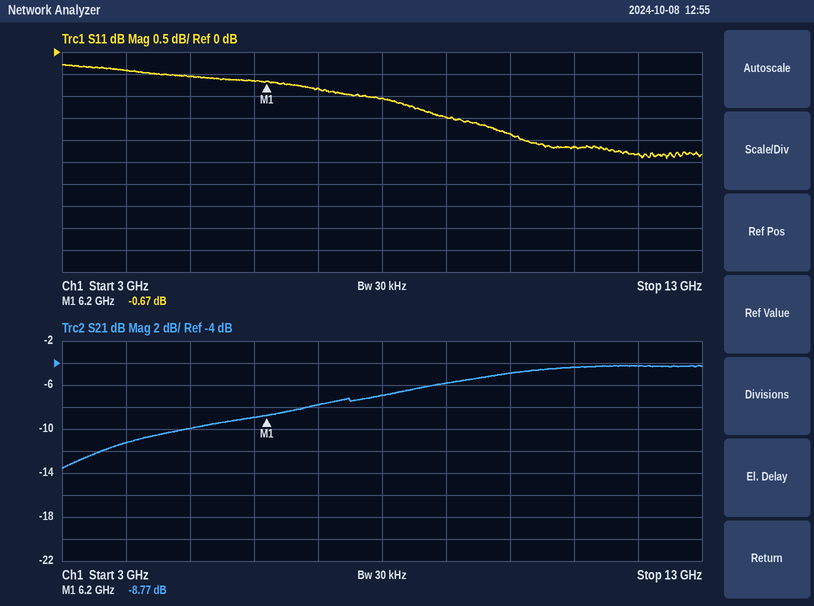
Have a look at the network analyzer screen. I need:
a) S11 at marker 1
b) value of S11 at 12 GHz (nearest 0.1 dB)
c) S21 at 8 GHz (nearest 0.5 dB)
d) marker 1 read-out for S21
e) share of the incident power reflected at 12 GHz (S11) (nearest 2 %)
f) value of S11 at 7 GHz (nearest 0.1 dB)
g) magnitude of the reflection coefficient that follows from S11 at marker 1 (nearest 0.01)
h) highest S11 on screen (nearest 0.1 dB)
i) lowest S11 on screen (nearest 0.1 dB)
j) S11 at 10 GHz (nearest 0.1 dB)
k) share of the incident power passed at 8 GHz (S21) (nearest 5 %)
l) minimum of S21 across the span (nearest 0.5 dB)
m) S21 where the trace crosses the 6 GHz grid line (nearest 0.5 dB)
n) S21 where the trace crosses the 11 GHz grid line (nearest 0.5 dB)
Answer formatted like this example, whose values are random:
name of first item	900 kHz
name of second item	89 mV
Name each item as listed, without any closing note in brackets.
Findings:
S11 at marker 1	-0.67 dB
value of S11 at 12 GHz	-2.3 dB
S21 at 8 GHz	-7.0 dB
marker 1 read-out for S21	-8.77 dB
share of the incident power reflected at 12 GHz (S11)	58 %
value of S11 at 7 GHz	-0.8 dB
magnitude of the reflection coefficient that follows from S11 at marker 1	0.93
highest S11 on screen	-0.3 dB
lowest S11 on screen	-2.4 dB
S11 at 10 GHz	-1.9 dB
share of the incident power passed at 8 GHz (S21)	20 %
minimum of S21 across the span	-13.5 dB
S21 where the trace crosses the 6 GHz grid line	-9.0 dB
S21 where the trace crosses the 11 GHz grid line	-4.5 dB
